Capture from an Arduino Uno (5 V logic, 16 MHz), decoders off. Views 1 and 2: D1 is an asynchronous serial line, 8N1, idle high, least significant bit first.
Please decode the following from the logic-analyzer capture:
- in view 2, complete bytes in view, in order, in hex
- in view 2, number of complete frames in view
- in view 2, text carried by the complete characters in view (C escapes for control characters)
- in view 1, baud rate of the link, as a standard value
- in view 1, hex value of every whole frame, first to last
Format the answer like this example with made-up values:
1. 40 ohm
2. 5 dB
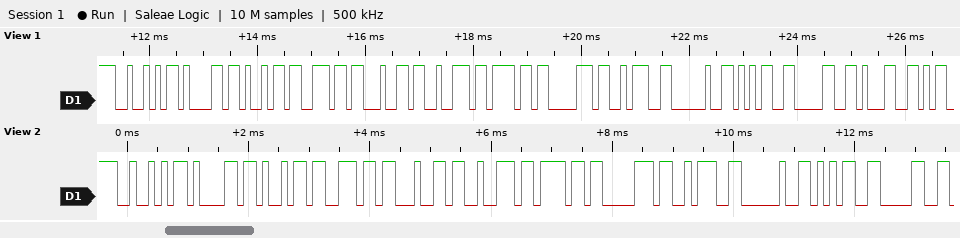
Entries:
1. 52 61 69 6E 64 72 6F 70 3A 20 35 30
2. 12
3. "Raindrop: 50"
4. 9600 baud
5. 0x52 0x61 0x69 0x6E 0x64 0x72 0x6F 0x70 0x3A 0x20 0x35 0x30 0x31
